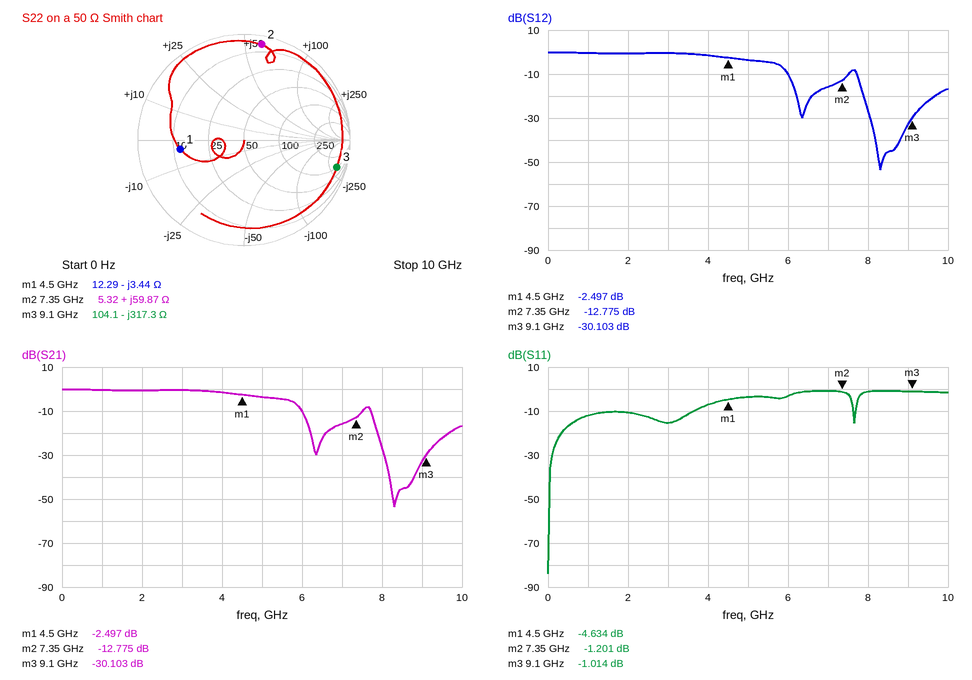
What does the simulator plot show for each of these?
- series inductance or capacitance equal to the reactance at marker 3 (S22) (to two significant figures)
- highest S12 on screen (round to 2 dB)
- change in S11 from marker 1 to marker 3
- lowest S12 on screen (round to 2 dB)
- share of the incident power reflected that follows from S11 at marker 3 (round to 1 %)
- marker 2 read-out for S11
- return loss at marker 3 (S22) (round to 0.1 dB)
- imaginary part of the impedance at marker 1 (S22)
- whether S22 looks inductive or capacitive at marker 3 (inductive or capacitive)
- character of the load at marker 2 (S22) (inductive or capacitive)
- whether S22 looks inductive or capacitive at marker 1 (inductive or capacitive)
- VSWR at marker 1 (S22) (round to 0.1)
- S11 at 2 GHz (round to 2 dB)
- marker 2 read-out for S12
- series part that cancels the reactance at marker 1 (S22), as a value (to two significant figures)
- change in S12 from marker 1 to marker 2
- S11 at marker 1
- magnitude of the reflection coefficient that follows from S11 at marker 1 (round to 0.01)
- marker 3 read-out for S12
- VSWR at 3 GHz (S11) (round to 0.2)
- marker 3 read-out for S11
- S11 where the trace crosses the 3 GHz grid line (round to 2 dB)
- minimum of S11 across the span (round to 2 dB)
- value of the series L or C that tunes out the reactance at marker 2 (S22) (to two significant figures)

55 fF
0 dB
3.620 dB
-54 dB
79 %
-1.201 dB
0.8 dB
-3.44 Ω
capacitive
inductive
capacitive
4.1
-10 dB
-12.775 dB
120 pH
-10.278 dB
-4.634 dB
0.59
-30.103 dB
1.4
-1.014 dB
-16 dB
-84 dB
360 fF
